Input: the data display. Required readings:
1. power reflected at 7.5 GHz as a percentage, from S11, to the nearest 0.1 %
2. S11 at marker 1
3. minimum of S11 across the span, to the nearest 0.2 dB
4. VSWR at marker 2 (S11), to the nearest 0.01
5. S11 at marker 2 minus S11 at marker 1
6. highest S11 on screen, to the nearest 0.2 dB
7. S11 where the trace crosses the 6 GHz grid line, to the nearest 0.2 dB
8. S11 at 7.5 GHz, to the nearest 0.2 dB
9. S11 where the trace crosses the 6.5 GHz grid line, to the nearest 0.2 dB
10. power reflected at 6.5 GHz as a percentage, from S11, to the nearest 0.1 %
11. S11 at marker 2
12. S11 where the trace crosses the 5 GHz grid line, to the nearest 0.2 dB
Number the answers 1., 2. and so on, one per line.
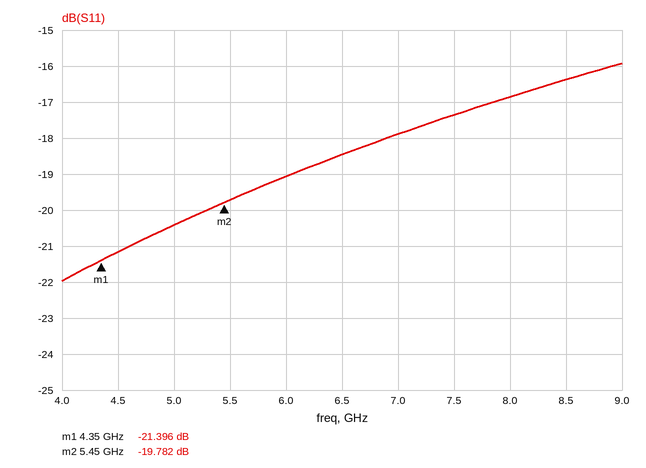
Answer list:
1. 1.8 %
2. -21.396 dB
3. -22.0 dB
4. 1.23
5. 1.614 dB
6. -16.0 dB
7. -19.0 dB
8. -17.4 dB
9. -18.4 dB
10. 1.4 %
11. -19.782 dB
12. -20.4 dB
